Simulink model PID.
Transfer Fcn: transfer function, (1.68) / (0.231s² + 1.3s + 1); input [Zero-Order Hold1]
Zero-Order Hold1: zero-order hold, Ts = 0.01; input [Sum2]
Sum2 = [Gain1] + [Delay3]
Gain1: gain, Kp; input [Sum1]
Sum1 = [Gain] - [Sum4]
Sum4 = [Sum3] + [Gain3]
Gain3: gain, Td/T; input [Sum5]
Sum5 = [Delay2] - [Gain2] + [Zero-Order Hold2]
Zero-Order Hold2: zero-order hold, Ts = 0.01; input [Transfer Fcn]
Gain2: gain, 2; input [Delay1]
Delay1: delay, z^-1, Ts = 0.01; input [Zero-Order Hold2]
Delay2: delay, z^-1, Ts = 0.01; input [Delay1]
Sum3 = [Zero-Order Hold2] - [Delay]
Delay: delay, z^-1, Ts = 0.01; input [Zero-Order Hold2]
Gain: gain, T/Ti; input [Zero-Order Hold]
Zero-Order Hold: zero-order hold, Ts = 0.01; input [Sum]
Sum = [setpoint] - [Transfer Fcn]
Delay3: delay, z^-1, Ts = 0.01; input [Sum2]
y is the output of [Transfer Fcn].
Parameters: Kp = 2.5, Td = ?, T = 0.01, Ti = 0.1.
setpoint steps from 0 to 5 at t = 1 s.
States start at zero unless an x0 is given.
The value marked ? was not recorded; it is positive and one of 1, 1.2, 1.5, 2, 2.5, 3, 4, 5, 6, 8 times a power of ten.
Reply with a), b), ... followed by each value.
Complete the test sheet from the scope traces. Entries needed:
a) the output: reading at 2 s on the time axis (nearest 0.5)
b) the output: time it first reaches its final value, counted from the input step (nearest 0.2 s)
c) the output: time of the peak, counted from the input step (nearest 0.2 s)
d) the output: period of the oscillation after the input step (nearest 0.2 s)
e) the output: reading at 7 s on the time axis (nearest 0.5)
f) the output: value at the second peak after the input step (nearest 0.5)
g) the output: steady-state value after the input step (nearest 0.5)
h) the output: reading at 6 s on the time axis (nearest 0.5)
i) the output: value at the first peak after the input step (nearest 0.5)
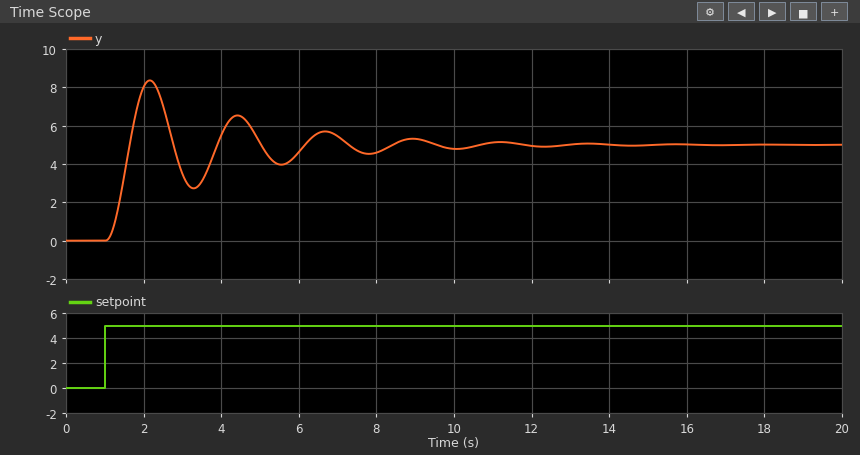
a) 8.0
b) 0.6 s
c) 1.2 s
d) 2.2 s
e) 5.5
f) 6.5
g) 5.0
h) 4.5
i) 8.5
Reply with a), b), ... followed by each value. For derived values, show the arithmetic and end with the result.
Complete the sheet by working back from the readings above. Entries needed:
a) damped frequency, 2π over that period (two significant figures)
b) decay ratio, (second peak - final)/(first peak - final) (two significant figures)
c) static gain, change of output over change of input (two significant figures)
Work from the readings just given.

a) 2π / 2.2 = 2.9 rad/s
b) (6.5 - 5) / (8.5 - 5) = 0.43
c) (5 - 0) / (5 - 0) = 1.0
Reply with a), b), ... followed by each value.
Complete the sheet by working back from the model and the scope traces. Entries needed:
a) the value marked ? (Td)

a) 1
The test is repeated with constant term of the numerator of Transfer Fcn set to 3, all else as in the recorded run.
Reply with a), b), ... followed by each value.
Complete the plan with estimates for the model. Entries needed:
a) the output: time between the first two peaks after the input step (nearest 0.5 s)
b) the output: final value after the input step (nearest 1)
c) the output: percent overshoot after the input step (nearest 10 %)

a) 2.0 s
b) 5
c) 60 %
